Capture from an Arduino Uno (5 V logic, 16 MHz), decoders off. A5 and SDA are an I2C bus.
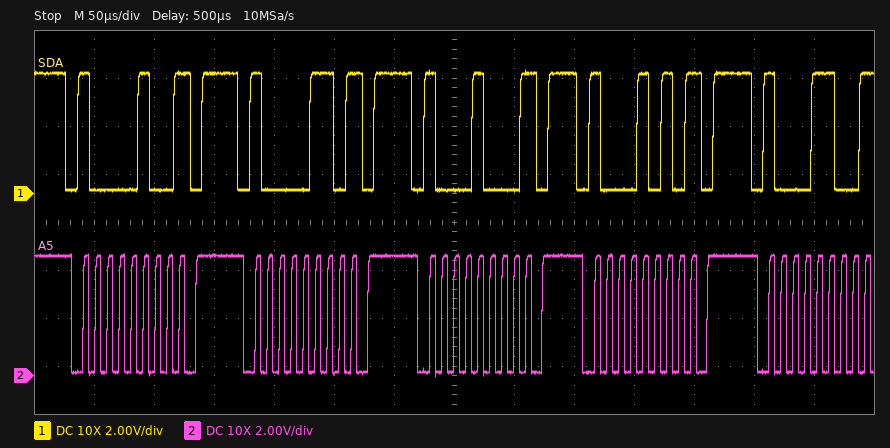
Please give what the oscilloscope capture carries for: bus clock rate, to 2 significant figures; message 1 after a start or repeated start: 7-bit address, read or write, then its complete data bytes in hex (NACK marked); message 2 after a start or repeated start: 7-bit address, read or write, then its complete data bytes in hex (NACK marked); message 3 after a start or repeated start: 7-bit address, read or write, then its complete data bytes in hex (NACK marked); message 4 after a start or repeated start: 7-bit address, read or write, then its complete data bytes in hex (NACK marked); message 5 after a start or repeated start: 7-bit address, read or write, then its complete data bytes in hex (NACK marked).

100 kHz
0x42 write NACK
0x43 write NACK
0x44 write NACK
0x45 write NACK
0x46 write NACK
